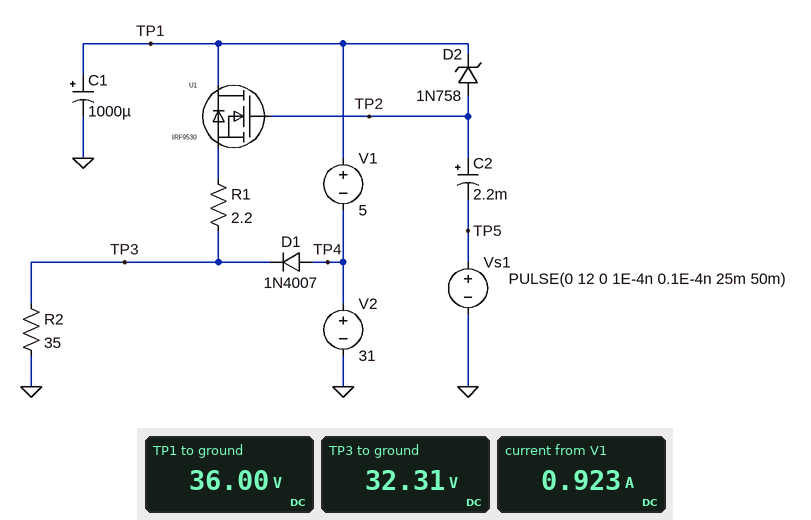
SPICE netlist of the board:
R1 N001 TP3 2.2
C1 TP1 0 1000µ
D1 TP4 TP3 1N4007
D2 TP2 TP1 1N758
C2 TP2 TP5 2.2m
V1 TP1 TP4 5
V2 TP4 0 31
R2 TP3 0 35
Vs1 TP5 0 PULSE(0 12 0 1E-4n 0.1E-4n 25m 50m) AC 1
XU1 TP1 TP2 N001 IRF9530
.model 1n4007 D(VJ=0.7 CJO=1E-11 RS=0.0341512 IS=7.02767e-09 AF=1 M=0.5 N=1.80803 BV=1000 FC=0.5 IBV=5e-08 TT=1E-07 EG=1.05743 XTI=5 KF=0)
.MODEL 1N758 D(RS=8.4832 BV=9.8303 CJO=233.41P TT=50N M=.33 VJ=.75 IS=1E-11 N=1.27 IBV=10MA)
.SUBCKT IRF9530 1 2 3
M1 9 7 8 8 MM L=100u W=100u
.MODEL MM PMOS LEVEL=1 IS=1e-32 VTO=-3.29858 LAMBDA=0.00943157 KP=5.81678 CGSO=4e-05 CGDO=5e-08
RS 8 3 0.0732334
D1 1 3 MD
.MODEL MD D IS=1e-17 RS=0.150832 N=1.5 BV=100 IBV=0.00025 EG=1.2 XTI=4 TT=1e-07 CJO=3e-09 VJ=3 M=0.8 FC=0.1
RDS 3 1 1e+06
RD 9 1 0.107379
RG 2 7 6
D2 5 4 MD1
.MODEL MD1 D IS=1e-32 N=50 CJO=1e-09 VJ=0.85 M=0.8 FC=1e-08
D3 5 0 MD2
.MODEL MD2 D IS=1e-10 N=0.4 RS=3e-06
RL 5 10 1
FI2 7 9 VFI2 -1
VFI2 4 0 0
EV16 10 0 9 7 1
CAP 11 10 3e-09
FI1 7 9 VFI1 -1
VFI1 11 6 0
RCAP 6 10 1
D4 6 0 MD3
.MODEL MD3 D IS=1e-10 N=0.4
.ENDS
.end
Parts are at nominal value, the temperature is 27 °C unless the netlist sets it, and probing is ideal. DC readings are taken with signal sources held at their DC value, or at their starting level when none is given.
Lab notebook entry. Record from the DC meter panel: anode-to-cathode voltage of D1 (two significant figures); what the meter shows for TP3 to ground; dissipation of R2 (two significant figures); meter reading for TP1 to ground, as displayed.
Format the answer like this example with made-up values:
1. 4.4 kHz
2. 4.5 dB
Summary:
1. -1.3 V
2. 32.31 V
3. 30 W
4. 36.00 V
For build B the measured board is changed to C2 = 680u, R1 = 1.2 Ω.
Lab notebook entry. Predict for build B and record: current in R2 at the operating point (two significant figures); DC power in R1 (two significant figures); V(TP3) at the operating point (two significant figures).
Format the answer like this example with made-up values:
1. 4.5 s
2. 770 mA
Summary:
1. 950 mA
2. 1.1 W
3. 33 V
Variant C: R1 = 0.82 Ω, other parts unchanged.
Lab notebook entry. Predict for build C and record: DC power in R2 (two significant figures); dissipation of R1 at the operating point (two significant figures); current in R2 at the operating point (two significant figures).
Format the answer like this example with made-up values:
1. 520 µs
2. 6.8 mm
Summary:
1. 32 W
2. 750 mW
3. 960 mA
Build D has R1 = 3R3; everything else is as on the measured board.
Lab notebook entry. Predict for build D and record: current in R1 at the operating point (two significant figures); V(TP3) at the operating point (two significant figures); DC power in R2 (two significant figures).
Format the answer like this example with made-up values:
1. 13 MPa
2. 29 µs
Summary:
1. 900 mA
2. 31 V
3. 28 W
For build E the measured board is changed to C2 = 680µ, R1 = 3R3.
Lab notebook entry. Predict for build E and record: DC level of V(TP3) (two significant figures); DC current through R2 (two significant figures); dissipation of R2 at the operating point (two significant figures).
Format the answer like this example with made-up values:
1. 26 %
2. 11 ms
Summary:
1. 31 V
2. 900 mA
3. 28 W
